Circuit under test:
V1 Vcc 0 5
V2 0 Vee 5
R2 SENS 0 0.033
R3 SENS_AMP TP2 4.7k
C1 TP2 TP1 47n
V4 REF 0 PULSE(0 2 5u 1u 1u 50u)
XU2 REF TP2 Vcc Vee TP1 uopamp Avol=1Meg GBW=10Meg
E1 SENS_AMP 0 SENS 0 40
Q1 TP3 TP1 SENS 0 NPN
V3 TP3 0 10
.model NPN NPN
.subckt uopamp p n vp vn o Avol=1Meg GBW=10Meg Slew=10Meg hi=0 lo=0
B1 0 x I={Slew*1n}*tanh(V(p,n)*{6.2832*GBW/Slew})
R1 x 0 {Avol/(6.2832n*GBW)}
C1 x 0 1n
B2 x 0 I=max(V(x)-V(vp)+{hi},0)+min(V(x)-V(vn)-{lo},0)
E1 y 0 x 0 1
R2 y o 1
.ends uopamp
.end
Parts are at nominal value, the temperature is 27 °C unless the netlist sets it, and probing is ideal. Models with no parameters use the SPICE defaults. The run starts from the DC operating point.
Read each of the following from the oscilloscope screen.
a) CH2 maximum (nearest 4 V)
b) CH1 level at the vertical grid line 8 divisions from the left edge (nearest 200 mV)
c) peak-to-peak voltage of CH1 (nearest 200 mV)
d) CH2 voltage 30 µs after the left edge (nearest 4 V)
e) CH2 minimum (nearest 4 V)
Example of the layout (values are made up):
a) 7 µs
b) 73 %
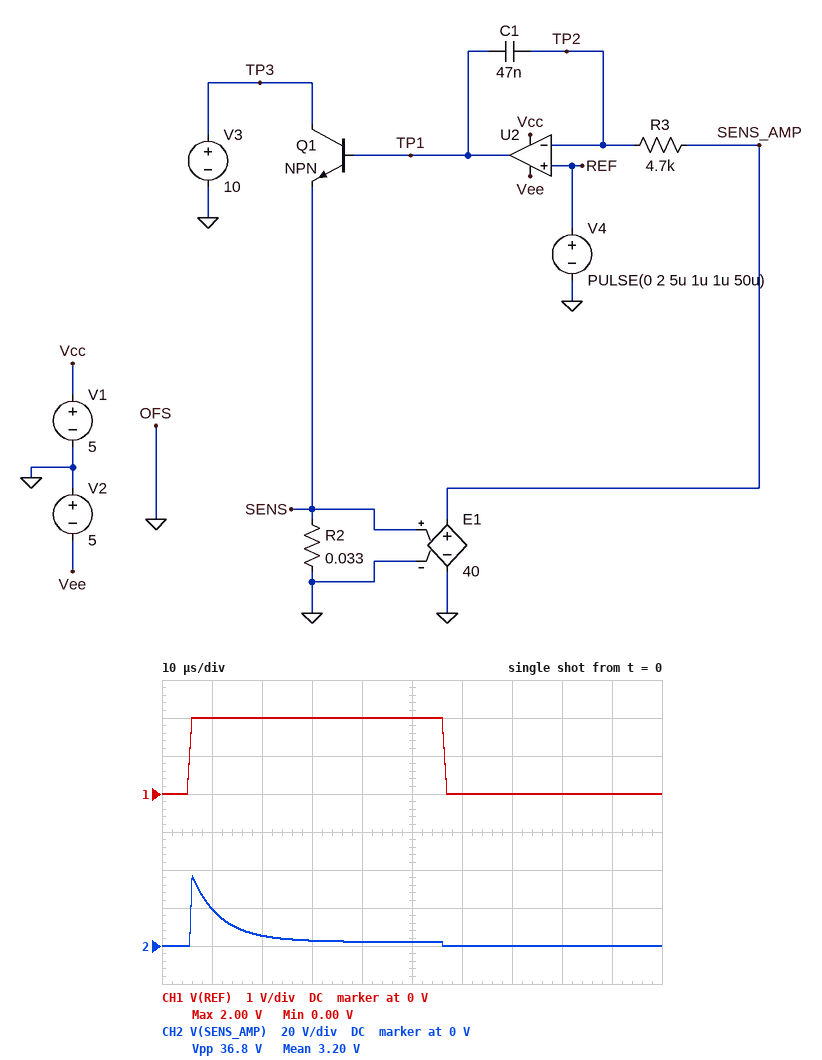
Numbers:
a) 36 V
b) 0 V
c) 2.0 V
d) 4 V
e) 0 V
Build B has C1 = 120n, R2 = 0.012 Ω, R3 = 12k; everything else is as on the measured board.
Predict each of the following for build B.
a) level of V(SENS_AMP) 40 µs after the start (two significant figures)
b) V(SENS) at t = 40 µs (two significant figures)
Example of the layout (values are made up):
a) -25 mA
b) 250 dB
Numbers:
a) 16 V
b) 410 mV
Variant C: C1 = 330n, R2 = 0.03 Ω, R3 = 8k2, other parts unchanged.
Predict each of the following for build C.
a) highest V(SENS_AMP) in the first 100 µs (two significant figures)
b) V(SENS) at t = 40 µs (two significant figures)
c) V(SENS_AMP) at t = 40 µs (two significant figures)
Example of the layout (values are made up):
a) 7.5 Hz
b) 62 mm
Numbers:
a) 38 V
b) 610 mV
c) 24 V
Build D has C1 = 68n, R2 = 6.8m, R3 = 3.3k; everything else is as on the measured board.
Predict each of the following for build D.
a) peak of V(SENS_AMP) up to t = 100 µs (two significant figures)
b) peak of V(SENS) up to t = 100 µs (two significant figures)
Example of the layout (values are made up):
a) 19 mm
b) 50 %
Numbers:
a) 35 V
b) 880 mV
